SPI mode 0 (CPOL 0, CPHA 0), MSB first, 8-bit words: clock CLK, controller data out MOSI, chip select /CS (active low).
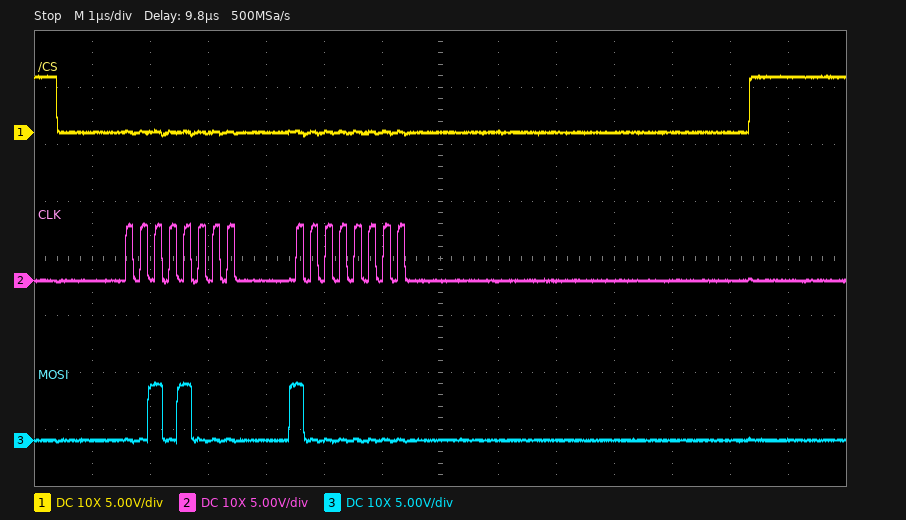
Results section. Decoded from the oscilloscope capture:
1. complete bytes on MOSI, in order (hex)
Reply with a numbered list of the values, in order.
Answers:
1. 0x28 0x80
